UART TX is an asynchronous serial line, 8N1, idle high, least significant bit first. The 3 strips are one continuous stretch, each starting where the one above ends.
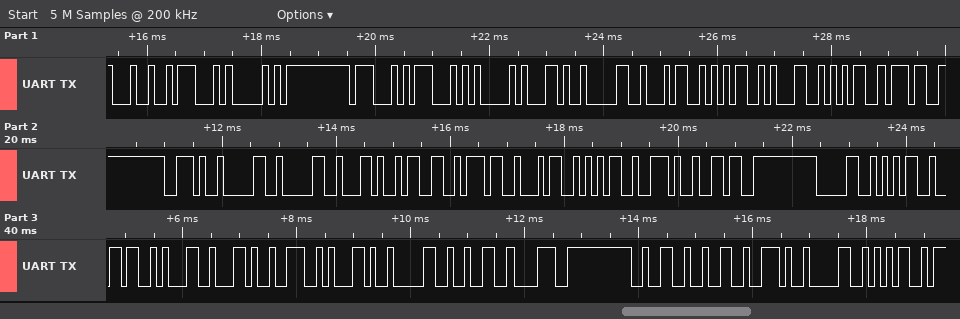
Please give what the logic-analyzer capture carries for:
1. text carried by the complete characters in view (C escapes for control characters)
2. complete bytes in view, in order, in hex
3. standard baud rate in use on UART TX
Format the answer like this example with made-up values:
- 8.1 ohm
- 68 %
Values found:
- "$GPGGA,045157.00,3745.60561,N,02822.05"
- 24 47 50 47 47 41 2C 30 34 35 31 35 37 2E 30 30 2C 33 37 34 35 2E 36 30 35 36 31 2C 4E 2C 30 32 38 32 32 2E 30 35
- 9600 baud
